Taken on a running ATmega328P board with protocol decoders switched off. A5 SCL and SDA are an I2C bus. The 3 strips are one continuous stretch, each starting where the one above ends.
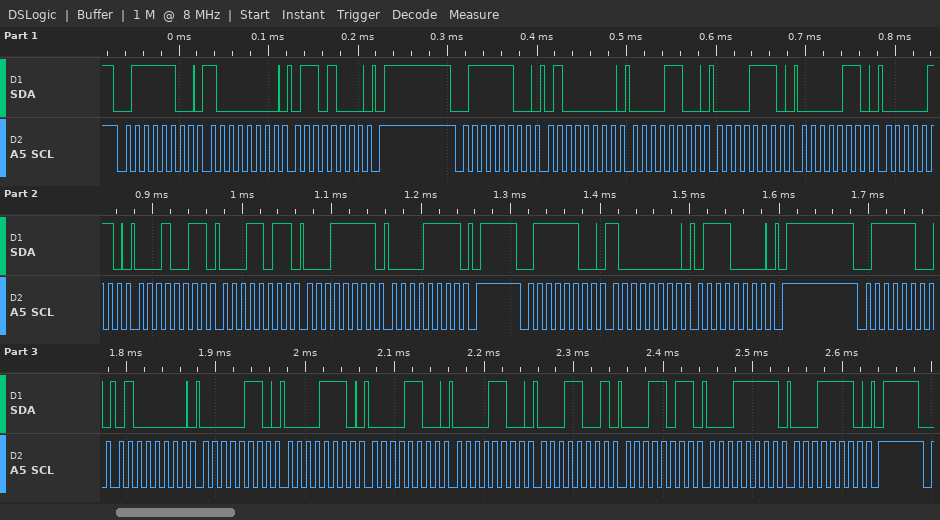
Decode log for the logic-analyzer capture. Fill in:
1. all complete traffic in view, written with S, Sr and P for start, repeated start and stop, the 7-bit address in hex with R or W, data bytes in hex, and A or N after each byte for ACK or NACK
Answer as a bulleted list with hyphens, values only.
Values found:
- S 3EW A 80 A 68 A P S 3EW A 40 A 0C A 0E A 06 A 06 A 13 A 1B A 1F A 0F A P S 3EW A 80 A 70 A P S 3EW A 40 A 06 A 0E A 0C A 0C A 19 A 1B A 1F A 1E A P
